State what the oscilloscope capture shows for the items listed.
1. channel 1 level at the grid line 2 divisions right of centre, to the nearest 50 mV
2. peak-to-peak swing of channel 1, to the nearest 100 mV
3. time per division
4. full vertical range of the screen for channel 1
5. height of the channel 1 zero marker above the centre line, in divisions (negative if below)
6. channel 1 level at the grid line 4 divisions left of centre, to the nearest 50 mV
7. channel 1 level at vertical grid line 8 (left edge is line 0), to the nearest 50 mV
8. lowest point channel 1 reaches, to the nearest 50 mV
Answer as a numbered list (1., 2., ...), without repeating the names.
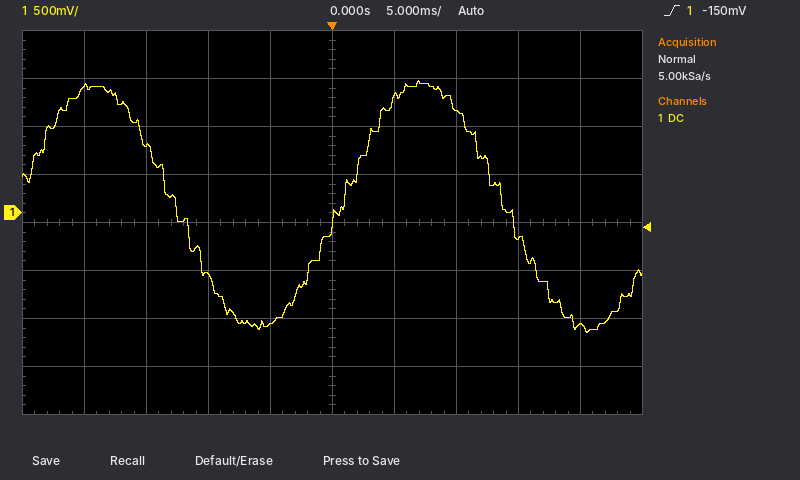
1. 1.05 V
2. 2.60 V
3. 5 ms
4. 4 V
5. +0.2 div
6. 1.30 V
7. -250 mV
8. -1.25 V
